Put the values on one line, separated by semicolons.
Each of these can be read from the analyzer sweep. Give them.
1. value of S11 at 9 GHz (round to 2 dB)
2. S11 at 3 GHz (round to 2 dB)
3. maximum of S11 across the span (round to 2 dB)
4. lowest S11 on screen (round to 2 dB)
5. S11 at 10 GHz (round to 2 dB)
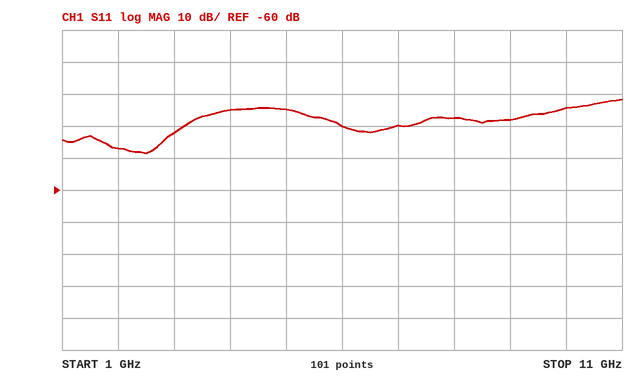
-38 dB; -42 dB; -32 dB; -48 dB; -34 dB
